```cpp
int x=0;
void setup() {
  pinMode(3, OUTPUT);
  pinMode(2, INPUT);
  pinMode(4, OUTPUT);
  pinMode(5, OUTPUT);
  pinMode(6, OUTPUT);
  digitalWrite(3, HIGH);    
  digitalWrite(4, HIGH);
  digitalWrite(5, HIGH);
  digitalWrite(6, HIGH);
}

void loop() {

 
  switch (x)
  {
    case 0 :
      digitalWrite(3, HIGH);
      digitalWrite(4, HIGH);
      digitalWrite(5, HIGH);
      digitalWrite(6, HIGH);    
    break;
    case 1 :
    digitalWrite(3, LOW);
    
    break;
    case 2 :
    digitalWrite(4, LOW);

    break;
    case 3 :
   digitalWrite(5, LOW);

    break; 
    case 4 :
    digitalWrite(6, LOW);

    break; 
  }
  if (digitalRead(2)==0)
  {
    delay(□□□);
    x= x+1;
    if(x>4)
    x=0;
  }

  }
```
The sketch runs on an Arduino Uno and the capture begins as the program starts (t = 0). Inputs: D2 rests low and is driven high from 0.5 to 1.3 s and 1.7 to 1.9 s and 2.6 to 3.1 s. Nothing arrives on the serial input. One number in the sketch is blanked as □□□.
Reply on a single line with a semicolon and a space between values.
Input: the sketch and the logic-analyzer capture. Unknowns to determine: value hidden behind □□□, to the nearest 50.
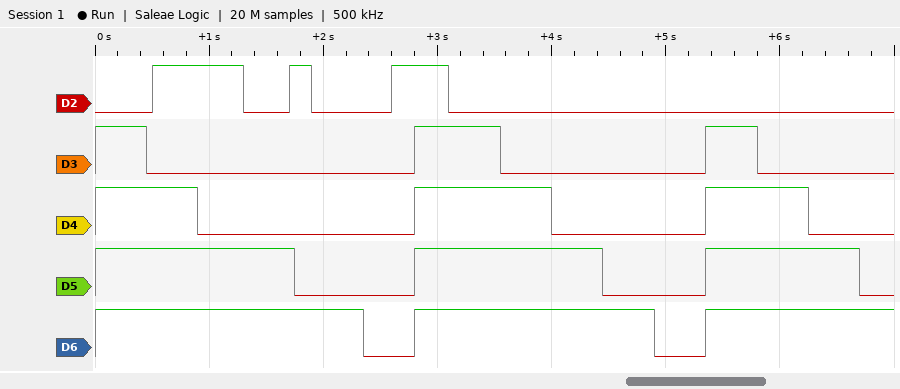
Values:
450
